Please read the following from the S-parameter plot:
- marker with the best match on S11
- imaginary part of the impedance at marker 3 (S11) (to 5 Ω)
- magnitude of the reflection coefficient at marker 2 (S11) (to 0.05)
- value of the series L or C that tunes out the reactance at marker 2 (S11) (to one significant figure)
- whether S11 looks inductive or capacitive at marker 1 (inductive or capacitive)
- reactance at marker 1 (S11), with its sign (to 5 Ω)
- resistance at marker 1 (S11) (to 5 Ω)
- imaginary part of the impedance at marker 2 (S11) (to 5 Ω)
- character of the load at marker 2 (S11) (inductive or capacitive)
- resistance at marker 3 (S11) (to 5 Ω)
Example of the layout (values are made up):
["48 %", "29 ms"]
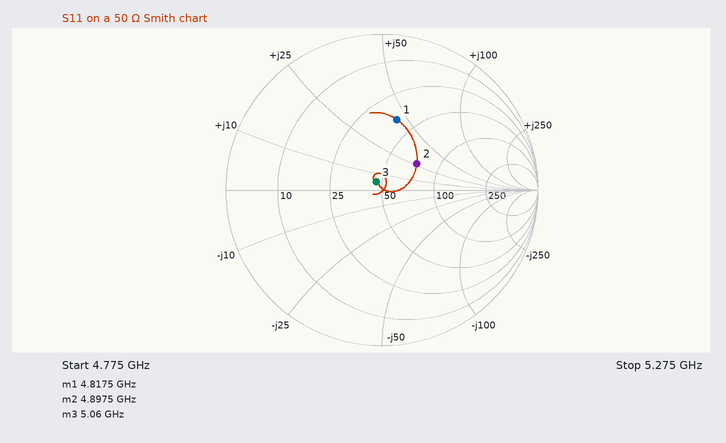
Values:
["marker 3", "+5 Ω", "0.30", "1 pF", "inductive", "+45 Ω", "40 Ω", "+25 Ω", "inductive", "45 Ω"]
